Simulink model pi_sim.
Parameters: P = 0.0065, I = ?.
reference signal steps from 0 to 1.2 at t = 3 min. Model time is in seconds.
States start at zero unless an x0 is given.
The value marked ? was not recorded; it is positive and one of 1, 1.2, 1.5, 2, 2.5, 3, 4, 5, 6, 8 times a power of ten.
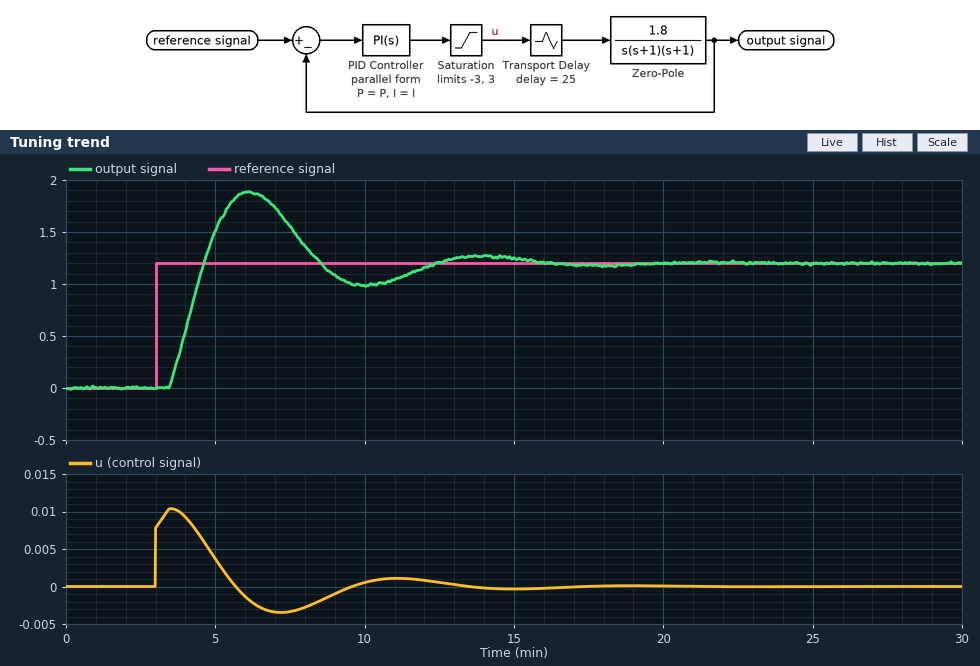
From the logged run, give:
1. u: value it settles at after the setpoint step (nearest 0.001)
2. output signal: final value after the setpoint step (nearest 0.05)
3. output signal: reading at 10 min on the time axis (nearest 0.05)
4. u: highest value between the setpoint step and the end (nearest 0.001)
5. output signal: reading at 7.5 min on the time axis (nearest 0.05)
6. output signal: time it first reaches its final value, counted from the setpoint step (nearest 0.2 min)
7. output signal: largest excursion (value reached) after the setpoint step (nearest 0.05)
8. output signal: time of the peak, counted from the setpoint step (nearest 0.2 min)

0.000
1.20
1.00
0.010
1.55
1.6 min
1.90
3.2 min
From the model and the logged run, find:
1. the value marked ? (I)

8e-05
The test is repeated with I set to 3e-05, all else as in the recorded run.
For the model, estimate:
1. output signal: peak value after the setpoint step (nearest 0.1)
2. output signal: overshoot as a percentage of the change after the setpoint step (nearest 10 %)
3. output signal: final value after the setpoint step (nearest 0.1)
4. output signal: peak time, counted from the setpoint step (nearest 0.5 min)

1.5
30 %
1.2
4.0 min
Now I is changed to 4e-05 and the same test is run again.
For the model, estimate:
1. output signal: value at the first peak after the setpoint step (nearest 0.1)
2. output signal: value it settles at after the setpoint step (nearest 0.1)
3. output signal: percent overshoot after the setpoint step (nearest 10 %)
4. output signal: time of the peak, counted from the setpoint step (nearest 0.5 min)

1.6
1.2
30 %
3.5 min
